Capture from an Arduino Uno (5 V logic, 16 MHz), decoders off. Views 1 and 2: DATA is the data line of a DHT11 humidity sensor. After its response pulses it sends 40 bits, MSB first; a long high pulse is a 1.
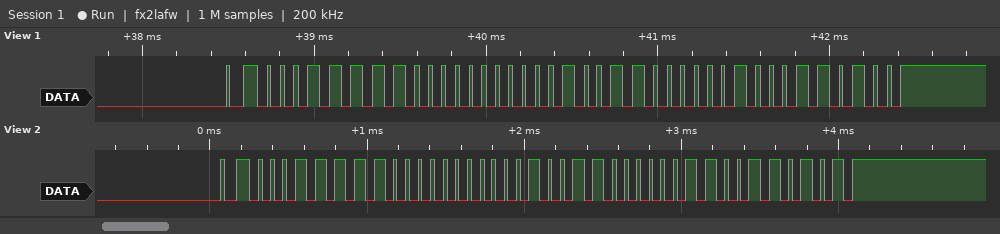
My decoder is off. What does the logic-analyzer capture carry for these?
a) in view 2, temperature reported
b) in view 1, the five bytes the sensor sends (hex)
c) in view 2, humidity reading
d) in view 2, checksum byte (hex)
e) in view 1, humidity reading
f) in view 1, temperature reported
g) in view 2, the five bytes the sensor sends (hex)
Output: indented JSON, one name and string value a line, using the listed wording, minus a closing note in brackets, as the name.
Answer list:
{
  "in view 2, temperature reported": "19.3 °C",
  "in view 1, the five bytes the sensor sends": "1F 00 13 02 34",
  "in view 2, humidity reading": "31 %",
  "in view 2, checksum byte": "0x35",
  "in view 1, humidity reading": "31 %",
  "in view 1, temperature reported": "19.2 °C",
  "in view 2, the five bytes the sensor sends": "1F 00 13 03 35"
}
